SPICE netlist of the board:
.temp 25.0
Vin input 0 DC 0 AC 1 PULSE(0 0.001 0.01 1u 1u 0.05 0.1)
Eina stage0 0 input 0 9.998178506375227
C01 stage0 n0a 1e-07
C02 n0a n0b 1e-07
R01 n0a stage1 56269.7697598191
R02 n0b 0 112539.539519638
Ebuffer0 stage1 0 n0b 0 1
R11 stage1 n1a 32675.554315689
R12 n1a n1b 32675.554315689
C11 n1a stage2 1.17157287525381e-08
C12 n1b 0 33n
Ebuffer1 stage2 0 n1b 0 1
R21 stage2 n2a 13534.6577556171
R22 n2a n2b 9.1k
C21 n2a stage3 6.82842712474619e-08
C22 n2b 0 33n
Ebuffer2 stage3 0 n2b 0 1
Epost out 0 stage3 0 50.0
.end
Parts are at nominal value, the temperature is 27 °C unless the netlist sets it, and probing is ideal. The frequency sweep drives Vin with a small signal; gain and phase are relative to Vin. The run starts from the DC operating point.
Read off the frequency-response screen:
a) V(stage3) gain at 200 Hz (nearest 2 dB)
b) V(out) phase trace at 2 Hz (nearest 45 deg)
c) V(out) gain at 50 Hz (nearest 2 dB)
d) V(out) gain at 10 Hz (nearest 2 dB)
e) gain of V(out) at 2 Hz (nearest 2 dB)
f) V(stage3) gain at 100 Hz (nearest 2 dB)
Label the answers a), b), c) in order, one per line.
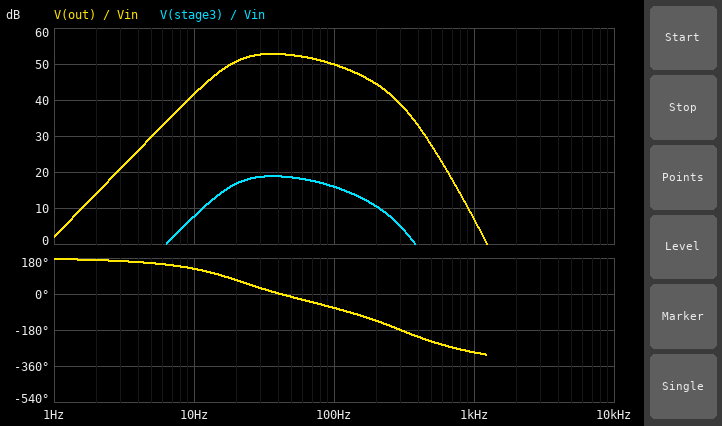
a) 10 dB
b) 180 deg
c) 52 dB
d) 42 dB
e) 14 dB
f) 16 dB
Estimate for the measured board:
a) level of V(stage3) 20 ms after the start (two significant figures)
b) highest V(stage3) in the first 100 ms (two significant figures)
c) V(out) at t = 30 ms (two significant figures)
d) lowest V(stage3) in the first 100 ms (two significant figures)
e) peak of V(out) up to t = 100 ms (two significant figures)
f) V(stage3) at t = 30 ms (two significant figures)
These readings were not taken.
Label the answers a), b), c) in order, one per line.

a) 1.3 mV
b) 5.5 mV
c) -99 mV
d) -5.5 mV
e) 280 mV
f) -2.0 mV
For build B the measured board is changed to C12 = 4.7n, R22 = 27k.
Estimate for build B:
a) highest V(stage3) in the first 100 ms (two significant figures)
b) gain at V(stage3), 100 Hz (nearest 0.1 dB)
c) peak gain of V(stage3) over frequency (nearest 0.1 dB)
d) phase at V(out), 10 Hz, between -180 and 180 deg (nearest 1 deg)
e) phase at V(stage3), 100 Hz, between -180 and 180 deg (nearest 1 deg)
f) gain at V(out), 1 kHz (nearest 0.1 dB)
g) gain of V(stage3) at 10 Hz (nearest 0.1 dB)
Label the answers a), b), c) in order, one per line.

a) 7.3 mV
b) 19.4 dB
c) 19.8 dB
d) 131 deg
e) -46 deg
f) 16.3 dB
g) 7.7 dB
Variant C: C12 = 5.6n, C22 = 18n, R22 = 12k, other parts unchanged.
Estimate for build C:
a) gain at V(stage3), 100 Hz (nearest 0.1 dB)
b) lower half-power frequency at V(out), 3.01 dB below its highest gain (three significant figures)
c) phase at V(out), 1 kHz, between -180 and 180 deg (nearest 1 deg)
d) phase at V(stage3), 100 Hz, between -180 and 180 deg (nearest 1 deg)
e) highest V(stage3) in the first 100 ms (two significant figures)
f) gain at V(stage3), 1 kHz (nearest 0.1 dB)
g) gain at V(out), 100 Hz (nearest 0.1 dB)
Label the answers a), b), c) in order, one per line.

a) 20.3 dB
b) 22.9 Hz
c) 77 deg
d) -14 deg
e) 9.9 mV
f) -6.7 dB
g) 54.3 dB
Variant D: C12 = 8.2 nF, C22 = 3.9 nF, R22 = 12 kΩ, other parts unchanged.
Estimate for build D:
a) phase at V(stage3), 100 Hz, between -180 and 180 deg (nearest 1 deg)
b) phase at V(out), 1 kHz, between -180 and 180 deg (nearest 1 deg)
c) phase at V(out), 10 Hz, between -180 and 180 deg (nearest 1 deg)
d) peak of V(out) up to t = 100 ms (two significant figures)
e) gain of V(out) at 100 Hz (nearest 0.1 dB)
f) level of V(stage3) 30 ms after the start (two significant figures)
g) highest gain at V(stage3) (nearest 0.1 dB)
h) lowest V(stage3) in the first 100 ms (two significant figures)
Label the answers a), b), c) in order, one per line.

a) -7 deg
b) 91 deg
c) 134 deg
d) 500 mV
e) 54.0 dB
f) -2.0 mV
g) 20.0 dB
h) -9.9 mV
